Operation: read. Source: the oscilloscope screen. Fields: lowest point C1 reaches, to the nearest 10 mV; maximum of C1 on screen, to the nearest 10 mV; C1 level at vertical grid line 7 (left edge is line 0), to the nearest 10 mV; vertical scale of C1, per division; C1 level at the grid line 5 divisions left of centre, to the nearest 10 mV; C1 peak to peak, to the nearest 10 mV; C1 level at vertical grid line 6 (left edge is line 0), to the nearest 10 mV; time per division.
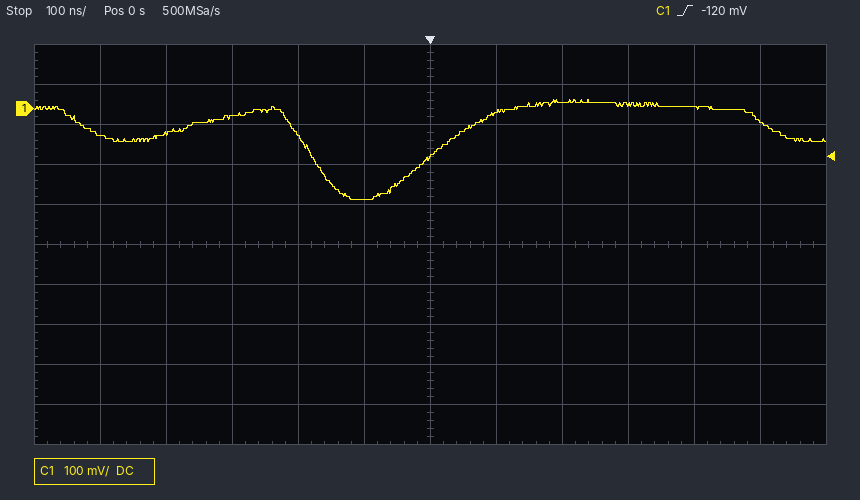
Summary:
-230 mV
20 mV
-10 mV
100 mV
-70 mV
250 mV
-120 mV
100 ns
